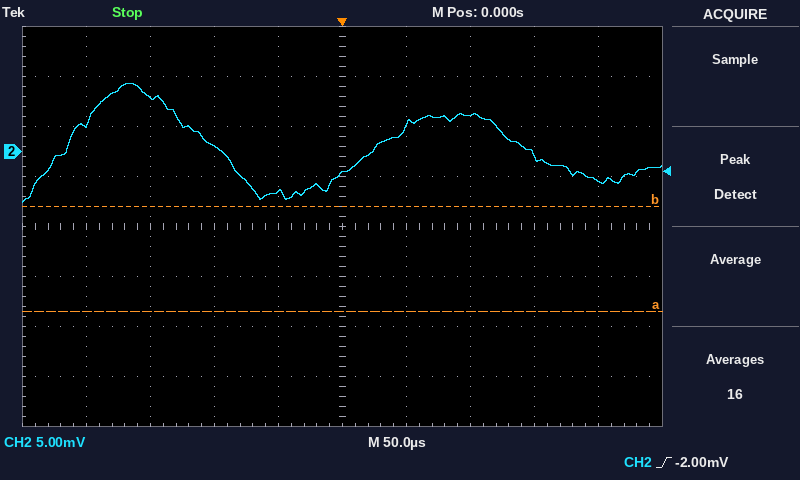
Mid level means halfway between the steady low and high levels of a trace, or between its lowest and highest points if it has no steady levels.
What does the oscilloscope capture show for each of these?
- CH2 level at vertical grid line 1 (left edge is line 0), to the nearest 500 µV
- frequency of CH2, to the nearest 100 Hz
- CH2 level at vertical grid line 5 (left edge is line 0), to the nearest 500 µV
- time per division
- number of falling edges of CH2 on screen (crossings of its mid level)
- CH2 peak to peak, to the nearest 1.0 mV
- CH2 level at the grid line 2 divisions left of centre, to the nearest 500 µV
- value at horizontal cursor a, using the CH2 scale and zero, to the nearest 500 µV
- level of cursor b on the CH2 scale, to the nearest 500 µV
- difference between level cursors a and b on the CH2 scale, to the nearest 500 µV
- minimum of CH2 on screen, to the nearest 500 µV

3.0 mV
4.1 kHz
-2.0 mV
50 µs
2
12.0 mV
500 µV
-16.0 mV
-5.5 mV
10.5 mV
-5.0 mV
